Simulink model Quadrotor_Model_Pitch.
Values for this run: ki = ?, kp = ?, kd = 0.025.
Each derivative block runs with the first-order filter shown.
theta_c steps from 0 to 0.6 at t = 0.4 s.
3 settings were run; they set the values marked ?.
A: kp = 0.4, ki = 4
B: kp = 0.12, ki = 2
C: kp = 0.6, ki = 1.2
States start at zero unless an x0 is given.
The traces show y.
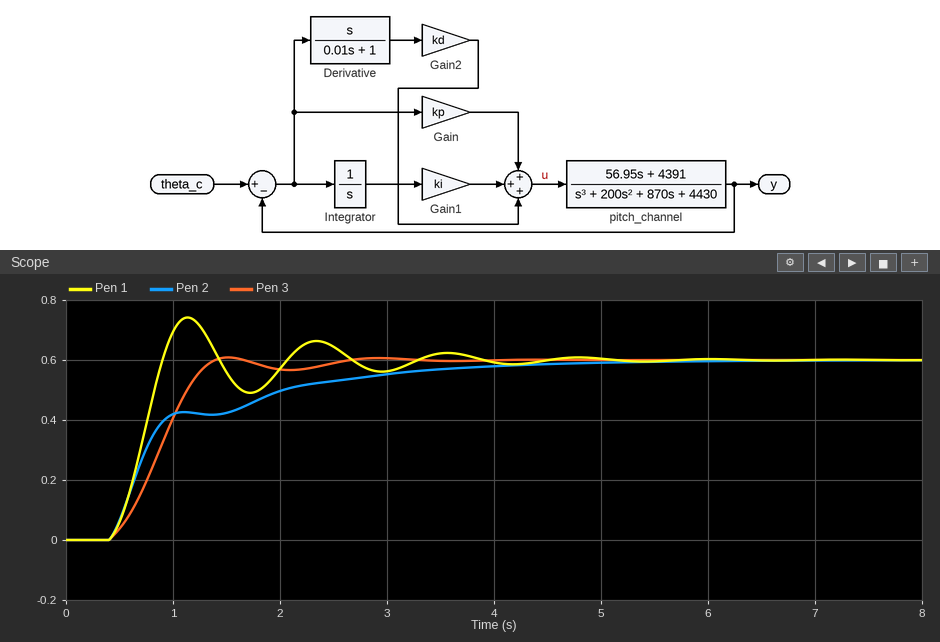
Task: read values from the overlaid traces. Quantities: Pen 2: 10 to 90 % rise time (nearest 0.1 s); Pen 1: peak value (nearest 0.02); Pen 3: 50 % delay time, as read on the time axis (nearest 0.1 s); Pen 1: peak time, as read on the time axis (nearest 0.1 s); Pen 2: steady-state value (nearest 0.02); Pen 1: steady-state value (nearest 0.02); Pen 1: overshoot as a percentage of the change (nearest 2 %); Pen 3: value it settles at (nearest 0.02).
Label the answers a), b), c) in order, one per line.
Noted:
a) 2.2 s
b) 0.74
c) 0.9 s
d) 1.1 s
e) 0.60
f) 0.60
g) 24 %
h) 0.60
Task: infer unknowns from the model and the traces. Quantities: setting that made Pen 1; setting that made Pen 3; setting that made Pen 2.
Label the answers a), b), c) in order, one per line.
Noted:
a) A
b) B
c) C
